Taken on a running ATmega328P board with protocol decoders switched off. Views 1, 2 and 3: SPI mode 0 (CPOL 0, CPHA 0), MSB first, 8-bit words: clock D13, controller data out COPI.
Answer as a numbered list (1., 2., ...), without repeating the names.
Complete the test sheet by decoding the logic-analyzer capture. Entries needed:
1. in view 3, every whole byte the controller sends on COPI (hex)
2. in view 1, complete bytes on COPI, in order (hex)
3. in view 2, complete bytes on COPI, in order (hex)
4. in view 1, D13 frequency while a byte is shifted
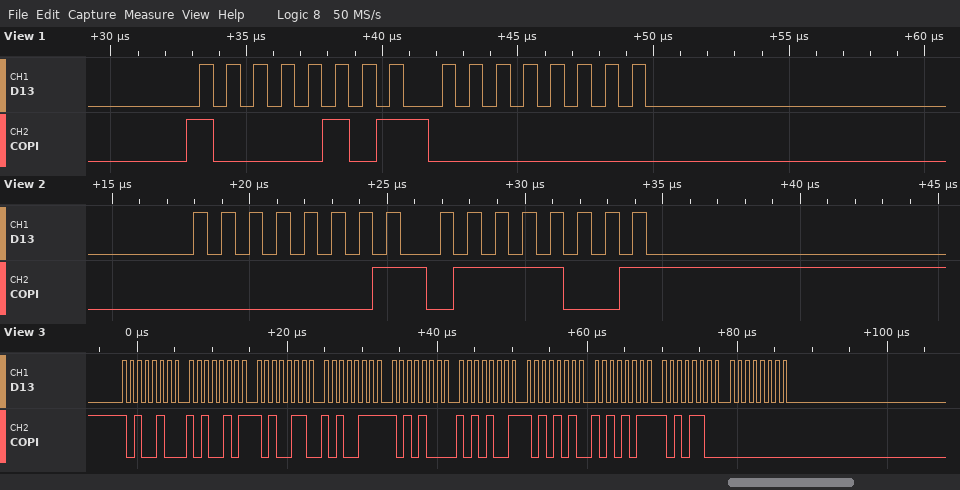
1. 0xA4 0xA5 0xA6 0xA7 0xA8 0xA9 0xAA 0xAB 0xAC 0x00
2. 85 00
3. 0x01 0x79
4. 1 MHz
